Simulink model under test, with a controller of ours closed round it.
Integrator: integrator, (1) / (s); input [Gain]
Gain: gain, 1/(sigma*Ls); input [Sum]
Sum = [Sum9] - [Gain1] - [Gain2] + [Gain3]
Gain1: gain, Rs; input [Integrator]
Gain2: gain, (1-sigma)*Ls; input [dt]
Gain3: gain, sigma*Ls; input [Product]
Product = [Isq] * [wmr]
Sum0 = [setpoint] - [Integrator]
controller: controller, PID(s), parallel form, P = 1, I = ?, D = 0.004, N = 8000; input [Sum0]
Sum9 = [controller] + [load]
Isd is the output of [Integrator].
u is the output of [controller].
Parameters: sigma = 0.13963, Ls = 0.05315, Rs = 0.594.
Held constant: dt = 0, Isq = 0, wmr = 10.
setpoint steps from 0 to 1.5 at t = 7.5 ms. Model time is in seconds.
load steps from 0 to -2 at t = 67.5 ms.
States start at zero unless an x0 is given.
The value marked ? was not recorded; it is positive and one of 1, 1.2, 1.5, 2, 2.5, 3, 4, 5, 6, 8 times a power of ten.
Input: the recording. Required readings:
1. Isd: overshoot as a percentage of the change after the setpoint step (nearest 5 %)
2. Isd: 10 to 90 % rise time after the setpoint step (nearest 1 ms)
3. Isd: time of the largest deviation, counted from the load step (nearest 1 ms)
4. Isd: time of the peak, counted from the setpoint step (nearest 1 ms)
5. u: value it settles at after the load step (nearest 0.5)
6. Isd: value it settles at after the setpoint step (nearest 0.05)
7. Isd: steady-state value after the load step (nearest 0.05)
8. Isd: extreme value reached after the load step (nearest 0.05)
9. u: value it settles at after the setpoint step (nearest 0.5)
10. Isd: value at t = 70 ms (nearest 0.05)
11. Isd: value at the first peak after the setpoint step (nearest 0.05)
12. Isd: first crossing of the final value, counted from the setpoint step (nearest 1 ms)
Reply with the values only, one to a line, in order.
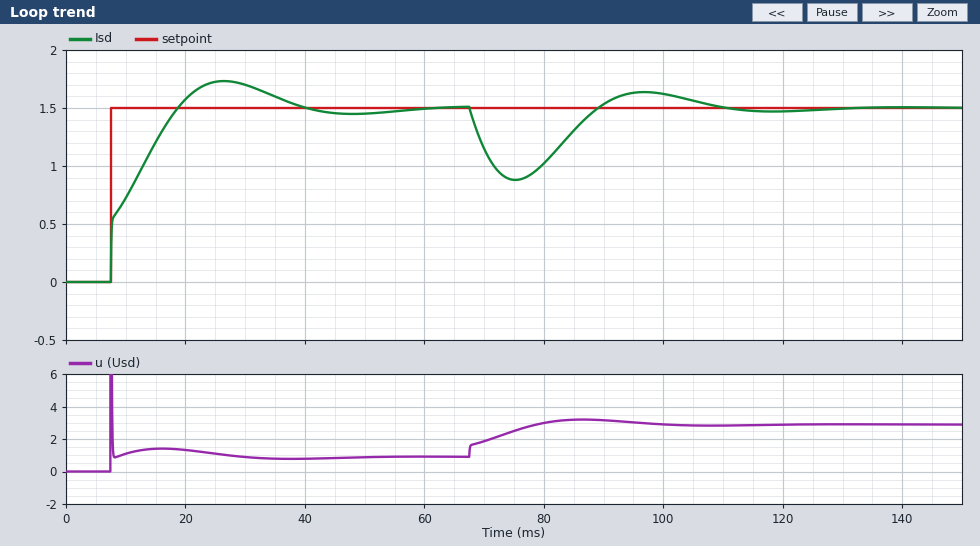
15 %
9 ms
8 ms
19 ms
3.0
1.50
1.50
0.90
1.0
1.15
1.75
11 ms
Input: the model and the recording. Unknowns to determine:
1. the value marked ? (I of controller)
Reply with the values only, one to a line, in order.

300
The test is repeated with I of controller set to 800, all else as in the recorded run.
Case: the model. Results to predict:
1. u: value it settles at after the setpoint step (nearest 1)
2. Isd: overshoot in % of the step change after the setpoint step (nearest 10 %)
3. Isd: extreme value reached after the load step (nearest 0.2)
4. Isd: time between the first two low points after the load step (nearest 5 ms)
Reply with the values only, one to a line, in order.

1
30 %
1.0
25 ms
